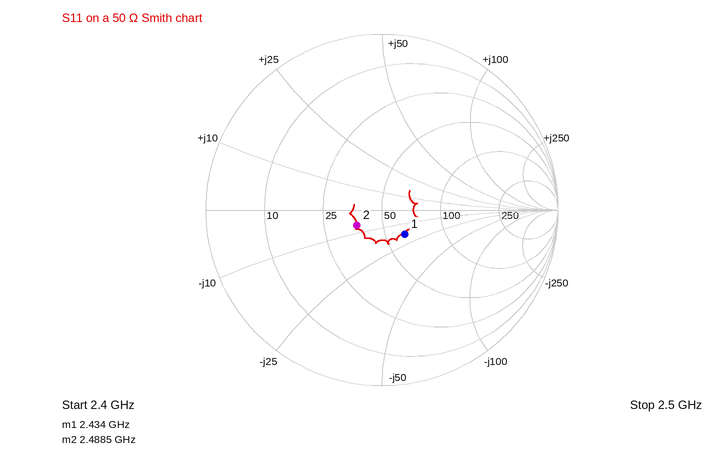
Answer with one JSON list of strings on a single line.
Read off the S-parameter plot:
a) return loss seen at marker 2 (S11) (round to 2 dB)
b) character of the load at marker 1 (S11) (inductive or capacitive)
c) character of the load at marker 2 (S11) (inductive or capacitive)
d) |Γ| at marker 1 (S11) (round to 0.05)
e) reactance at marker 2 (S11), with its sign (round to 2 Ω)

["16 dB", "capacitive", "capacitive", "0.20", "-6 Ω"]
